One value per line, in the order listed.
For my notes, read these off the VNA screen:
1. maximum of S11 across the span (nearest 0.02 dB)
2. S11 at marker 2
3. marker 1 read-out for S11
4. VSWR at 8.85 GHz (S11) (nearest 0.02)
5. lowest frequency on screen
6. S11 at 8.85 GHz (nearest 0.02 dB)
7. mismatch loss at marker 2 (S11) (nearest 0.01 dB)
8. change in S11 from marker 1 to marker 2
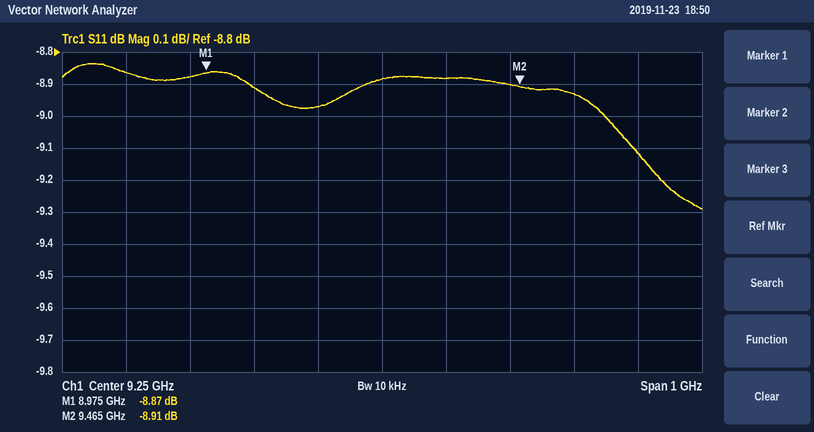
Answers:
-8.84 dB
-8.91 dB
-8.87 dB
2.12
8.75 GHz
-8.86 dB
0.60 dB
-0.04 dB
